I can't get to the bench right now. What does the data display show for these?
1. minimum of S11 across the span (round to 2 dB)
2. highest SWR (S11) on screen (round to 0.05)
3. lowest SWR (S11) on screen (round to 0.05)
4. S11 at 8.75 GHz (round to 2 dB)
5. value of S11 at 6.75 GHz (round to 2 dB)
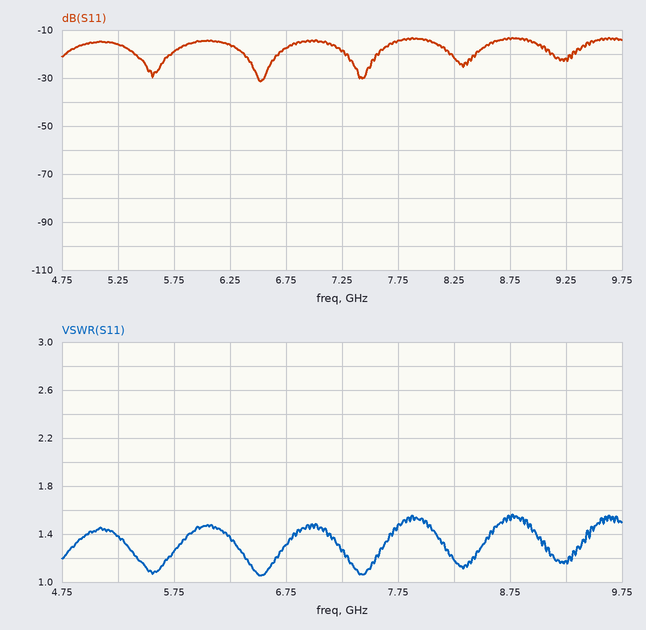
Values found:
-32 dB
1.55
1.05
-14 dB
-18 dB
